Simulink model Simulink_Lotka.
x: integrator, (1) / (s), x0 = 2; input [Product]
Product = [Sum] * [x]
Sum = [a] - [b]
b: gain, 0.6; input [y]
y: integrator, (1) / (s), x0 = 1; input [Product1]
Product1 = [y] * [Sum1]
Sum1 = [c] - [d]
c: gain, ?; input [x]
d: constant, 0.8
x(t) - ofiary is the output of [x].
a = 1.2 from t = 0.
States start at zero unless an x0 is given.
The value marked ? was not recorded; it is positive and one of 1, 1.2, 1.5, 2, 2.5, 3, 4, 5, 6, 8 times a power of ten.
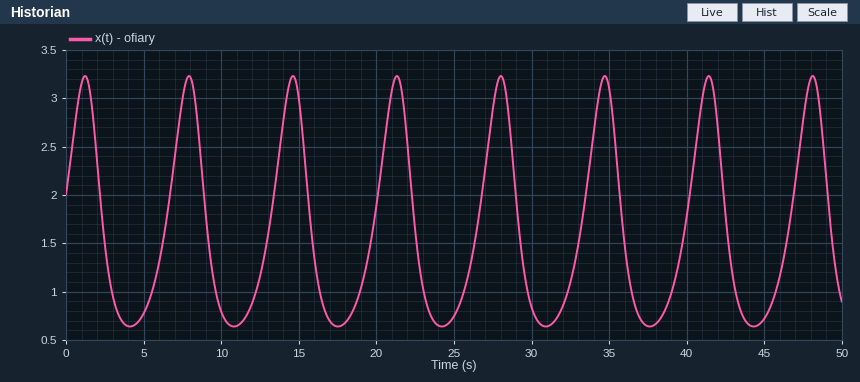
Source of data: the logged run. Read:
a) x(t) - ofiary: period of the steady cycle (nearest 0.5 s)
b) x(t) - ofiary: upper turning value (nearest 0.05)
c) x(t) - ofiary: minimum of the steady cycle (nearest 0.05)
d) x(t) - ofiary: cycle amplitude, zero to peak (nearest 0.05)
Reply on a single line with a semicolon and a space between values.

6.5 s; 3.25; 0.65; 1.30
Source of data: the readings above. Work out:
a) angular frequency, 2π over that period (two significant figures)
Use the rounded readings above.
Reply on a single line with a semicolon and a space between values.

0.97 rad/s
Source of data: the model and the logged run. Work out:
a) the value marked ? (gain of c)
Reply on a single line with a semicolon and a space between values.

0.5
